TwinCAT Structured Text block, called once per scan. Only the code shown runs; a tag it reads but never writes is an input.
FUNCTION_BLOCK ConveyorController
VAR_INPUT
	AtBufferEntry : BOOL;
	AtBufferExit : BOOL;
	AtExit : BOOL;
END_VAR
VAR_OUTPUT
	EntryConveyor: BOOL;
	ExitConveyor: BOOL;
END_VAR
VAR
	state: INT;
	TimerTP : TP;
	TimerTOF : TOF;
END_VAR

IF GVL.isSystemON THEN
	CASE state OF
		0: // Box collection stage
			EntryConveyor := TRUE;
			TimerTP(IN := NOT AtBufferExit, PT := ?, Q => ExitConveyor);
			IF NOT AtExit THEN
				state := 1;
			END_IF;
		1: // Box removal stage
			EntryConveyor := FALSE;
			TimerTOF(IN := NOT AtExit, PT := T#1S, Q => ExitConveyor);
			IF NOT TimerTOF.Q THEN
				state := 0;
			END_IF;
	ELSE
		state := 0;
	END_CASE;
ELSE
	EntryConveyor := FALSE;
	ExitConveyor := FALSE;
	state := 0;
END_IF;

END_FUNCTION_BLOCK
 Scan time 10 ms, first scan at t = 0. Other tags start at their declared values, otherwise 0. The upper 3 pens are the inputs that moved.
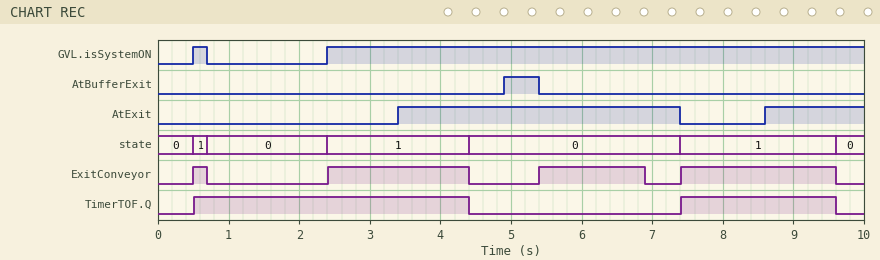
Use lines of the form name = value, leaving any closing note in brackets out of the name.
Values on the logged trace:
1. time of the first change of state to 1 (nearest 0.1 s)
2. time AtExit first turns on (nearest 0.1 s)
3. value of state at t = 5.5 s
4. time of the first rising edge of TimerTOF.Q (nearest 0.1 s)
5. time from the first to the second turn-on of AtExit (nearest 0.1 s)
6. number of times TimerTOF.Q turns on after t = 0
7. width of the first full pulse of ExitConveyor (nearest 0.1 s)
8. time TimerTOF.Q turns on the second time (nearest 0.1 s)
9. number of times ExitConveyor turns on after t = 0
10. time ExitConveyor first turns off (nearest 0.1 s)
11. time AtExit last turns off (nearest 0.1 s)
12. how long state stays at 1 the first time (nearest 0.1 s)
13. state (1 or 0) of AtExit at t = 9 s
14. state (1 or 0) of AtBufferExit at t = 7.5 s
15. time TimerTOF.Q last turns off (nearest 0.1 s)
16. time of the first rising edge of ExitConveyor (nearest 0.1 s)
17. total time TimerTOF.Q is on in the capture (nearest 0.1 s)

time of the first change of state to 1 = 0.5 s
time AtExit first turns on = 3.4 s
value of state at t = 5.5 s = 0
time of the first rising edge of TimerTOF.Q = 0.5 s
time from the first to the second turn-on of AtExit = 5.2 s
number of times TimerTOF.Q turns on after t = 0 = 2
width of the first full pulse of ExitConveyor = 0.2 s
time TimerTOF.Q turns on the second time = 7.4 s
number of times ExitConveyor turns on after t = 0 = 4
time ExitConveyor first turns off = 0.7 s
time AtExit last turns off = 7.4 s
how long state stays at 1 the first time = 0.2 s
state (1 or 0) of AtExit at t = 9 s = 1
state (1 or 0) of AtBufferExit at t = 7.5 s = 0
time TimerTOF.Q last turns off = 9.6 s
time of the first rising edge of ExitConveyor = 0.5 s
total time TimerTOF.Q is on in the capture = 6.1 s
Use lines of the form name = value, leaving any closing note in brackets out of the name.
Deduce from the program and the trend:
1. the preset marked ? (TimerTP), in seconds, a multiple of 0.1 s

the preset marked ? (TimerTP), in seconds, a multiple of 0.1 s = 1.5 s
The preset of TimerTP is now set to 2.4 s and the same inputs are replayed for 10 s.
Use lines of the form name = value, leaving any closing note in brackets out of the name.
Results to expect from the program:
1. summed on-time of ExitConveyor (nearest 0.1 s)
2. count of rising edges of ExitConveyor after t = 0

summed on-time of ExitConveyor = 6.4 s
count of rising edges of ExitConveyor after t = 0 = 3
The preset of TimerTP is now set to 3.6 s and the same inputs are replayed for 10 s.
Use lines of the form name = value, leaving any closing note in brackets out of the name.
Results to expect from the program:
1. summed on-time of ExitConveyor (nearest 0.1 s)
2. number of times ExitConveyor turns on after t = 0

summed on-time of ExitConveyor = 6.4 s
number of times ExitConveyor turns on after t = 0 = 3
